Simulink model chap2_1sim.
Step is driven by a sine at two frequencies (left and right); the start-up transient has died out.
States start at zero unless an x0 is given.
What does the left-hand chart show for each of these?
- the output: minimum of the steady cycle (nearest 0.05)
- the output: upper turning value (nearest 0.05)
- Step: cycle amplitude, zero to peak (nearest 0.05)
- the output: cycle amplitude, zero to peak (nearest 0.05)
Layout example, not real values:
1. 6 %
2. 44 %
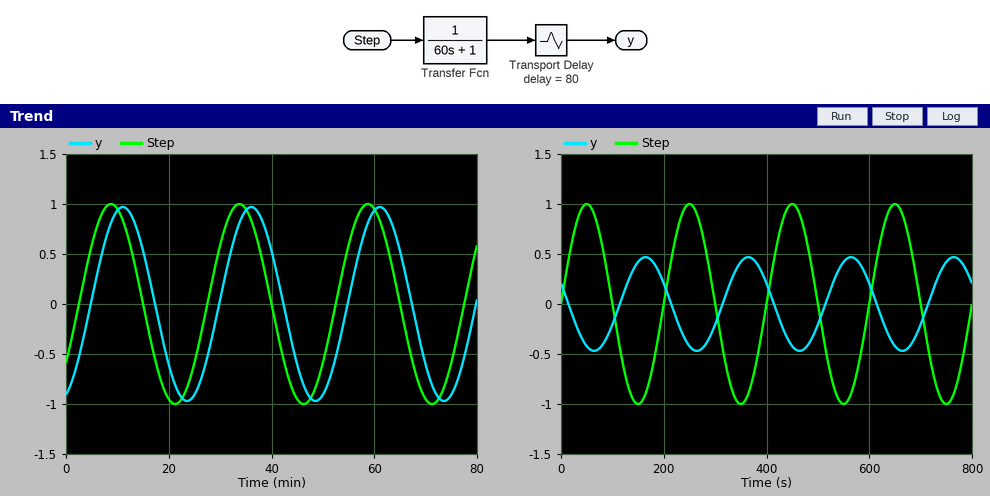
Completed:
1. -0.95
2. 0.95
3. 1.00
4. 0.95
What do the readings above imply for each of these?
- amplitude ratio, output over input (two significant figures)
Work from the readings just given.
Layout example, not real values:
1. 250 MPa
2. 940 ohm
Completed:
1. 0.95
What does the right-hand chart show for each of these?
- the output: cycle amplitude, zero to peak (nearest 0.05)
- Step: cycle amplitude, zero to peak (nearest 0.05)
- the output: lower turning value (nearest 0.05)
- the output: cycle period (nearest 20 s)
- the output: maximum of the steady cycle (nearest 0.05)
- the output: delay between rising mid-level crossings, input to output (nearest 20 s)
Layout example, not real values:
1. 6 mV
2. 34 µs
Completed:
1. 0.45
2. 1.00
3. -0.45
4. 200 s
5. 0.45
6. 120 s
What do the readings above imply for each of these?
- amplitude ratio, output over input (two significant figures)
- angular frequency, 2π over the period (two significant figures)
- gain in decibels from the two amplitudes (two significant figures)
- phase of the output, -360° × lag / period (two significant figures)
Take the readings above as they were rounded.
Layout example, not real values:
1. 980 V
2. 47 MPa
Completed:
1. 0.45
2. 0.031 rad/s
3. -6.9 dB
4. -220°
